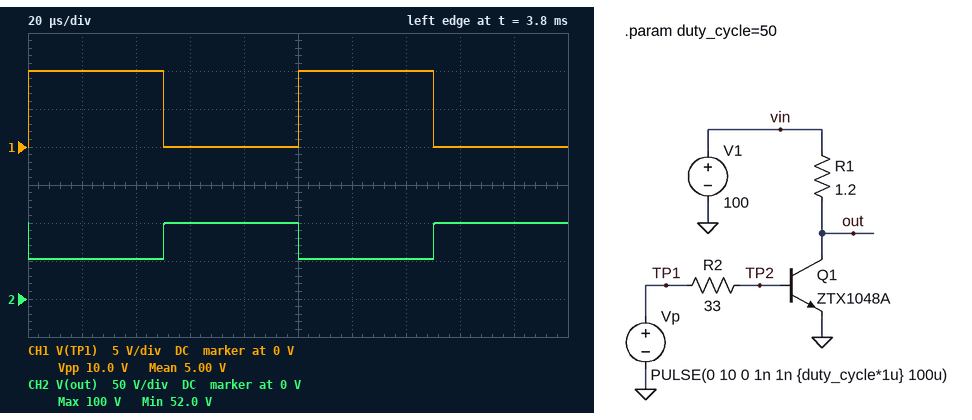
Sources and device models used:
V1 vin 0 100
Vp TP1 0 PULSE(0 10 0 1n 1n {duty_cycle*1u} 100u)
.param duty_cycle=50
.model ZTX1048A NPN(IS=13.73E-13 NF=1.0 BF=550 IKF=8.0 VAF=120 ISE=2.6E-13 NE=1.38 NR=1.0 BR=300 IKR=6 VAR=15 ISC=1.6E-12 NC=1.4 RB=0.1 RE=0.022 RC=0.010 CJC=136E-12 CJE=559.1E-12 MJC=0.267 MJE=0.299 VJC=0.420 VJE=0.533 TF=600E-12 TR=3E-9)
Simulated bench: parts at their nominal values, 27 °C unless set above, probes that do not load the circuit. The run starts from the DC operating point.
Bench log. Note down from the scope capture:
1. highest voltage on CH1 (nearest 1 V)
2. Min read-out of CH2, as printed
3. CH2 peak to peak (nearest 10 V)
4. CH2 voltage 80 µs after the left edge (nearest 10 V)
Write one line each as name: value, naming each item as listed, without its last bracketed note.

highest voltage on CH1: 10 V
Min read-out of CH2, as printed: 52.0 V
CH2 peak to peak: 50 V
CH2 voltage 80 µs after the left edge: 100 V
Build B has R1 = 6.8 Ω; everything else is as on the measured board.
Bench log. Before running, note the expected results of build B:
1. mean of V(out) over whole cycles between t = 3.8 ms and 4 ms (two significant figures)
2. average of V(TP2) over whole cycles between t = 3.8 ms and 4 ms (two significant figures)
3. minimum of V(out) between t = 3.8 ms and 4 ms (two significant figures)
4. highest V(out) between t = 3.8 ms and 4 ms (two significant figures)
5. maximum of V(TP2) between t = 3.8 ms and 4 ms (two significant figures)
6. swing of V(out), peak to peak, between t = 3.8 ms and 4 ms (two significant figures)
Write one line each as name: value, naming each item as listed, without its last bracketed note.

mean of V(out) over whole cycles between t = 3.8 ms and 4 ms: 50 V
average of V(TP2) over whole cycles between t = 3.8 ms and 4 ms: 600 mV
minimum of V(out) between t = 3.8 ms and 4 ms: 500 mV
highest V(out) between t = 3.8 ms and 4 ms: 100 V
maximum of V(TP2) between t = 3.8 ms and 4 ms: 1.2 V
swing of V(out), peak to peak, between t = 3.8 ms and 4 ms: 100 V
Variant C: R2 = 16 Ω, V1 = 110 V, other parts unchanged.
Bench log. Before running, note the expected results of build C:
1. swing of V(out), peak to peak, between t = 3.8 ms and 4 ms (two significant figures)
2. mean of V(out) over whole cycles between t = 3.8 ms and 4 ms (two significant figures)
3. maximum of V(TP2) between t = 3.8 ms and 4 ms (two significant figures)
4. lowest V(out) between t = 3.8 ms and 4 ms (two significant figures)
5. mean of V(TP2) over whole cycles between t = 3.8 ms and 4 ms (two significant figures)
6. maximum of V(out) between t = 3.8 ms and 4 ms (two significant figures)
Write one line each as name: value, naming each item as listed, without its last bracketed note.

swing of V(out), peak to peak, between t = 3.8 ms and 4 ms: 66 V
mean of V(out) over whole cycles between t = 3.8 ms and 4 ms: 77 V
maximum of V(TP2) between t = 3.8 ms and 4 ms: 2.1 V
lowest V(out) between t = 3.8 ms and 4 ms: 44 V
mean of V(TP2) over whole cycles between t = 3.8 ms and 4 ms: 1.1 V
maximum of V(out) between t = 3.8 ms and 4 ms: 110 V
